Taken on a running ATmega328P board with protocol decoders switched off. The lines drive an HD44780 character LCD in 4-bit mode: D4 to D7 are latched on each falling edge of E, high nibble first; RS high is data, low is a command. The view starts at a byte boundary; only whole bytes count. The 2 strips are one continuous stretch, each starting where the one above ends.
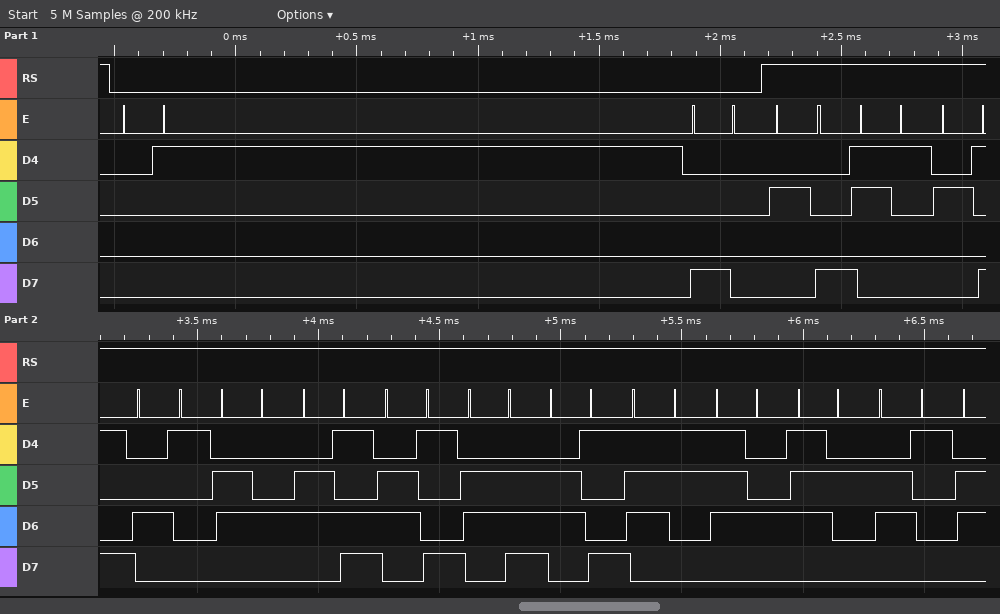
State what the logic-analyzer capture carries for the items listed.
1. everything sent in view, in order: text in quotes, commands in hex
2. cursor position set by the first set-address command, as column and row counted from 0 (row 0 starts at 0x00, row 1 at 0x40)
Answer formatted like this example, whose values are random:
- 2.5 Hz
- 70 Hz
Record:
- 0x01 0x80 "(1)Administra"
- column 0, row 0
